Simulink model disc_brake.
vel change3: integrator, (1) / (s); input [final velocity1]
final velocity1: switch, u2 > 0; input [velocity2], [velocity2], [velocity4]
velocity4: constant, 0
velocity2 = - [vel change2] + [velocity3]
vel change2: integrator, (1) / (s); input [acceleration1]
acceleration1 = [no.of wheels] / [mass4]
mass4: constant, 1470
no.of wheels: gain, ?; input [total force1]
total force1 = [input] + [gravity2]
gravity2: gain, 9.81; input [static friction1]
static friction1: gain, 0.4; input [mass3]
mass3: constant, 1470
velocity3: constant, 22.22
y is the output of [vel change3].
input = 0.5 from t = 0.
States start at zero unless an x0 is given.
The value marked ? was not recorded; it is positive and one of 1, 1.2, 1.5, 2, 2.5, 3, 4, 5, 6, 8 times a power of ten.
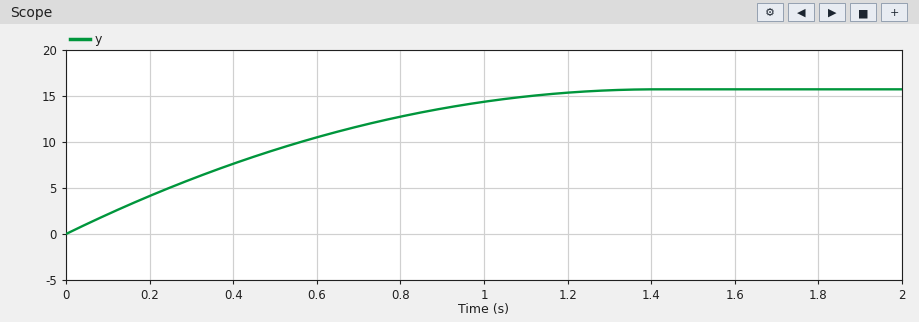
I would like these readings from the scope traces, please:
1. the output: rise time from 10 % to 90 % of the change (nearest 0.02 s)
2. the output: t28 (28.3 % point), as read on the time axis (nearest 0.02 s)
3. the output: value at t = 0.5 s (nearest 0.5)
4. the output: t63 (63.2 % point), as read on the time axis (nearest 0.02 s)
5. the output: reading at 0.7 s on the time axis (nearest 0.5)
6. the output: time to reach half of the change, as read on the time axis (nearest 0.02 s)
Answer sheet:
0.90 s
0.22 s
9.0
0.56 s
11.5
0.42 s
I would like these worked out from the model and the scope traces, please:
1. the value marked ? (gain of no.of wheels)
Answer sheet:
4
